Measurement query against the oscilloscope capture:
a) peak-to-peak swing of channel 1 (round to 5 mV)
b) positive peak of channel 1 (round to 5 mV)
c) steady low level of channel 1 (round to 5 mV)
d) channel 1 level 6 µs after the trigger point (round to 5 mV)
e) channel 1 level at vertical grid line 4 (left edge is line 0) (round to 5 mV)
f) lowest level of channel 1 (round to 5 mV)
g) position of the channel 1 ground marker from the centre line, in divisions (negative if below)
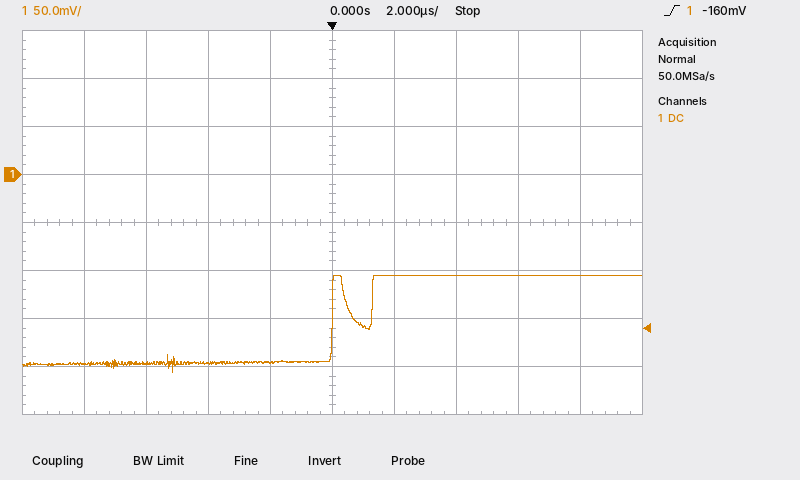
100 mV
-105 mV
-195 mV
-105 mV
-195 mV
-205 mV
+1.0 div
